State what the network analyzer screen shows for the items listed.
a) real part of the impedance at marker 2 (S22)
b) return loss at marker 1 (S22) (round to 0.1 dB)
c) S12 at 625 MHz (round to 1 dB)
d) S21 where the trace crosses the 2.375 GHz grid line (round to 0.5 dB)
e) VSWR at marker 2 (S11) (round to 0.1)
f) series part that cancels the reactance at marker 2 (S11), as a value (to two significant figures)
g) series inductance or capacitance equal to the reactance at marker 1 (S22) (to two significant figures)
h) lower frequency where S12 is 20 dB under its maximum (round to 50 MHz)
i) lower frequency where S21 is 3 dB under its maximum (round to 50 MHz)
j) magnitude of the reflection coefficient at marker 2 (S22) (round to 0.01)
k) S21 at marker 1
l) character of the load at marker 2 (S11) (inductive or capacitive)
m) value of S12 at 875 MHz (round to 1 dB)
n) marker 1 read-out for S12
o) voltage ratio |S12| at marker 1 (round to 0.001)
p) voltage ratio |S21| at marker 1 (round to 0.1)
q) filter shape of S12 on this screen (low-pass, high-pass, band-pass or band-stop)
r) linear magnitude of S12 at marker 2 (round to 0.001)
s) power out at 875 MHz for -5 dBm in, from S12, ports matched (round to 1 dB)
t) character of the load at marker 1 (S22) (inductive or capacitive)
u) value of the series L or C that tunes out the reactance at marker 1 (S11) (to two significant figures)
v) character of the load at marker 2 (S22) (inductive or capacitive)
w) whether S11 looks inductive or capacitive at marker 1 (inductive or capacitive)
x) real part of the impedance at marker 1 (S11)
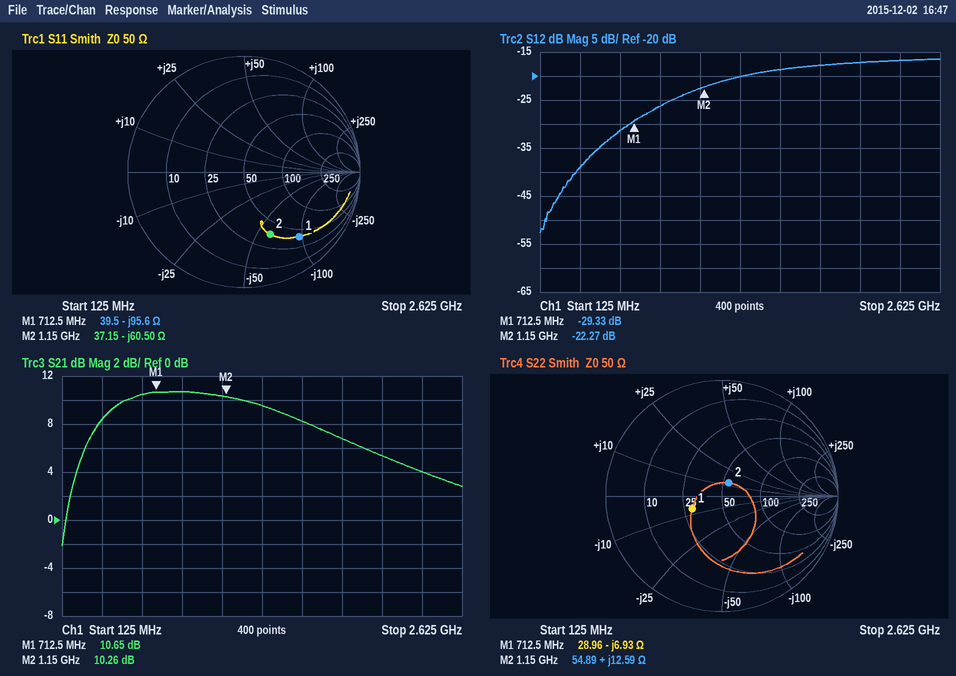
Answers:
54.89 Ω
11.1 dB
-31 dB
4.0 dB
3.8
8.4 nH
32 pF
450 MHz
350 MHz
0.13
10.65 dB
capacitive
-26 dB
-29.33 dB
0.034
3.4
high-pass
0.077
-31 dBm
capacitive
21 nH
inductive
capacitive
39.5 Ω
